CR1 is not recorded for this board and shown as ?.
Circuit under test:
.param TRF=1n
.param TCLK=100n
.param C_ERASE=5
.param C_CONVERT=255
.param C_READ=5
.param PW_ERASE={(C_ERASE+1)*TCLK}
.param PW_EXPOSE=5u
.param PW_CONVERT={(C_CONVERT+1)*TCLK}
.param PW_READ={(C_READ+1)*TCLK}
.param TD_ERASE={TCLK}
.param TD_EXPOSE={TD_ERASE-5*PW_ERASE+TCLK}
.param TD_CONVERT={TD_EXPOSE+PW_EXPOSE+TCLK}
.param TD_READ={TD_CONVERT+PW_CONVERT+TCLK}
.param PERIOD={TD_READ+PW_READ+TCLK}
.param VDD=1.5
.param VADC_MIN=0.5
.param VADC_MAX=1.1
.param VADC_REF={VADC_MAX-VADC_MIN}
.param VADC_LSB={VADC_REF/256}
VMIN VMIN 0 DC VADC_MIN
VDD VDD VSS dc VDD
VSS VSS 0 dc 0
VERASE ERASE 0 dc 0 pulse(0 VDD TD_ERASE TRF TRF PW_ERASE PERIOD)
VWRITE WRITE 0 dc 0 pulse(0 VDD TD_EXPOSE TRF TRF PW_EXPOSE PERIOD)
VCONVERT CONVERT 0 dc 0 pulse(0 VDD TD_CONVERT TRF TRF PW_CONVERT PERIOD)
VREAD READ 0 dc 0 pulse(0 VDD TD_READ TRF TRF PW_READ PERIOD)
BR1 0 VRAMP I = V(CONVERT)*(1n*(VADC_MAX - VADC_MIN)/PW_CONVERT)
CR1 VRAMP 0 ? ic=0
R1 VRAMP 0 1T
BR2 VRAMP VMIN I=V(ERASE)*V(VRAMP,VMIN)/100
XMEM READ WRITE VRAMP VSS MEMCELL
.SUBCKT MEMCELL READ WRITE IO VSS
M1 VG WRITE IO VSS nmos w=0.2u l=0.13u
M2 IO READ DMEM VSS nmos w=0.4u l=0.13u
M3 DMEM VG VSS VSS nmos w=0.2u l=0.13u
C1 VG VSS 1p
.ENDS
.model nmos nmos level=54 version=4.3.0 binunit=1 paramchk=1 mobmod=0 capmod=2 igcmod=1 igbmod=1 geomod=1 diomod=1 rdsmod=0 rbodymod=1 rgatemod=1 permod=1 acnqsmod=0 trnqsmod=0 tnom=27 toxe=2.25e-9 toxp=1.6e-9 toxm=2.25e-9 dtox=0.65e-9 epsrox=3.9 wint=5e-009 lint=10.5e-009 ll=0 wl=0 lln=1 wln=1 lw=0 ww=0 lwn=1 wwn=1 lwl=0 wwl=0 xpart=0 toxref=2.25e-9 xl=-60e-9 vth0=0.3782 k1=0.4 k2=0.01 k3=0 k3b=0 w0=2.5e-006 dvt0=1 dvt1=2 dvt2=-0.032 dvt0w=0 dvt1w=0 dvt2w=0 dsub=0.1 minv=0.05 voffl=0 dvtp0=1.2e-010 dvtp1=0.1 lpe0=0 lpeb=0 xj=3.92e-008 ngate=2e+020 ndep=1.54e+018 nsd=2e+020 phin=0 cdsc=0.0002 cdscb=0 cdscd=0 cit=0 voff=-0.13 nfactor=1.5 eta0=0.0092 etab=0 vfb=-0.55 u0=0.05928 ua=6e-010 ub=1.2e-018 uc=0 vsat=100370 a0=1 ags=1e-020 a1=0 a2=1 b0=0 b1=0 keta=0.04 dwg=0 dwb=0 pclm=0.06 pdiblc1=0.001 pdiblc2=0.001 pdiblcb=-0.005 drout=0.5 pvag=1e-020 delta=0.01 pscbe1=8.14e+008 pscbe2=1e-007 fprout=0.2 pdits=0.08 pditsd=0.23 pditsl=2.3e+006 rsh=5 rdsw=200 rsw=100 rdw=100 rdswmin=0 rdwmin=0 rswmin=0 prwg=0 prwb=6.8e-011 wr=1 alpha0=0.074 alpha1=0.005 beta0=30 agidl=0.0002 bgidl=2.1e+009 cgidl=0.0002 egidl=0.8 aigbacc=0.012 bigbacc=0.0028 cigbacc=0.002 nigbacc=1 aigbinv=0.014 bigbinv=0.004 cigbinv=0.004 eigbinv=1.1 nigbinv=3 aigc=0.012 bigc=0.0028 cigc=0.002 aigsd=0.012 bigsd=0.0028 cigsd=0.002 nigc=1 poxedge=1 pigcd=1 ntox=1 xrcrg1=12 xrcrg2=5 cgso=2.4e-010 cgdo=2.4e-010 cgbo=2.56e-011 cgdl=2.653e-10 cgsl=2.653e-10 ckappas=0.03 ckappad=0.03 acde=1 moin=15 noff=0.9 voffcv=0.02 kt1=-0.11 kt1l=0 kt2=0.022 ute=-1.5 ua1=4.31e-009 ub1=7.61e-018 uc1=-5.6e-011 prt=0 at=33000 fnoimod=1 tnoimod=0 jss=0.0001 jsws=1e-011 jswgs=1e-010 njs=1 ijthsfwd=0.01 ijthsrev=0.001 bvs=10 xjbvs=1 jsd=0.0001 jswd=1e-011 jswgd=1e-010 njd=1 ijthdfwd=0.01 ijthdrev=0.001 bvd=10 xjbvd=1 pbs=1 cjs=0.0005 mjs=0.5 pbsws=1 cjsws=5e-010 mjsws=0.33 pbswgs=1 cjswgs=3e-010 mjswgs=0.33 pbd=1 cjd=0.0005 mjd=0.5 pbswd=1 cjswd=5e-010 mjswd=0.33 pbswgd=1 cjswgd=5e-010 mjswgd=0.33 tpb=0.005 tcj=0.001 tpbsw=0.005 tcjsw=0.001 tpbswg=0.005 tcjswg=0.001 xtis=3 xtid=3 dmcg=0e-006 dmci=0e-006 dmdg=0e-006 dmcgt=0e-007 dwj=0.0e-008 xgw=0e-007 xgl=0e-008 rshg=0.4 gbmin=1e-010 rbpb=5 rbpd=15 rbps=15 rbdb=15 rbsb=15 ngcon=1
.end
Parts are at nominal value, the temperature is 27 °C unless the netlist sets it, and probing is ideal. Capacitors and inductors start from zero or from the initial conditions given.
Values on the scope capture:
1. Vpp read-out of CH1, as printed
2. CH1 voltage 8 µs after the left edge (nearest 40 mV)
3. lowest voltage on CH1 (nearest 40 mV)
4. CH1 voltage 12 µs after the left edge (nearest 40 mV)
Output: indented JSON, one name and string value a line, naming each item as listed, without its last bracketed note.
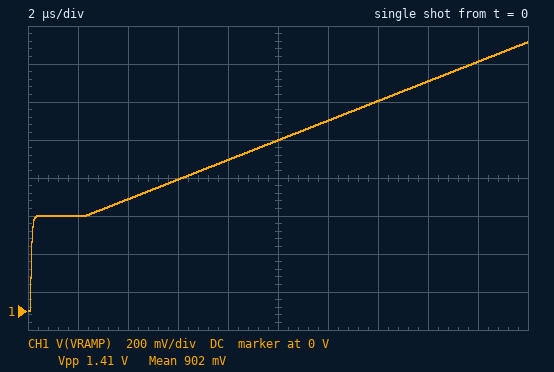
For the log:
{
  "Vpp read-out of CH1, as printed": "1.41 V",
  "CH1 voltage 8 µs after the left edge": "800 mV",
  "lowest voltage on CH1": "0 V",
  "CH1 voltage 12 µs after the left edge": "1.00 V"
}
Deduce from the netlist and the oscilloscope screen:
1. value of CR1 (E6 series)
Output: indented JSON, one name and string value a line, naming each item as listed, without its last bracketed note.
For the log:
{
  "value of CR1": "680 pF"
}
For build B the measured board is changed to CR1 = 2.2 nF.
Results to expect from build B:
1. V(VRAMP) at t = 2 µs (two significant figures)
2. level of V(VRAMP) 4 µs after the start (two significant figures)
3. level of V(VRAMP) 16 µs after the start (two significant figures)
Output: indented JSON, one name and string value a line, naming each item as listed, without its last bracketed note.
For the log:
{
  "V(VRAMP) at t = 2 µs": "490 mV",
  "level of V(VRAMP) 4 µs after the start": "520 mV",
  "level of V(VRAMP) 16 µs after the start": "710 mV"
}
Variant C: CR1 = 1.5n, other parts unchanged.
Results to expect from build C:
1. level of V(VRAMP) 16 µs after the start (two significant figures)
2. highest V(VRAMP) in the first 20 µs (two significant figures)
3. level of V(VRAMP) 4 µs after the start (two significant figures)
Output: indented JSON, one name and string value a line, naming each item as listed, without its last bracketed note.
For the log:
{
  "level of V(VRAMP) 16 µs after the start": "820 mV",
  "highest V(VRAMP) in the first 20 µs": "910 mV",
  "level of V(VRAMP) 4 µs after the start": "540 mV"
}
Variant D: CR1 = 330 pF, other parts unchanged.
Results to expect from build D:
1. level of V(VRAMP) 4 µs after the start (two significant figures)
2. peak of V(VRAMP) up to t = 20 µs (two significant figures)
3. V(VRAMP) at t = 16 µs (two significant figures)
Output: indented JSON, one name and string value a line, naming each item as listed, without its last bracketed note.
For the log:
{
  "level of V(VRAMP) 4 µs after the start": "680 mV",
  "peak of V(VRAMP) up to t = 20 µs": "2.4 V",
  "V(VRAMP) at t = 16 µs": "2.0 V"
}
